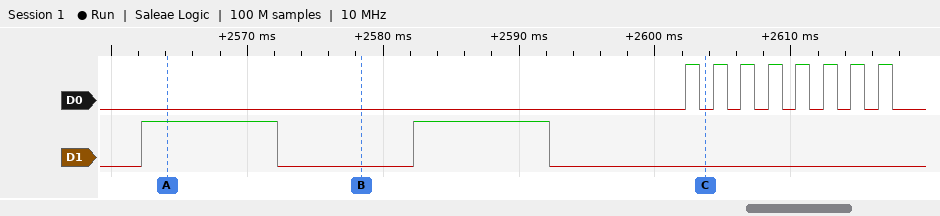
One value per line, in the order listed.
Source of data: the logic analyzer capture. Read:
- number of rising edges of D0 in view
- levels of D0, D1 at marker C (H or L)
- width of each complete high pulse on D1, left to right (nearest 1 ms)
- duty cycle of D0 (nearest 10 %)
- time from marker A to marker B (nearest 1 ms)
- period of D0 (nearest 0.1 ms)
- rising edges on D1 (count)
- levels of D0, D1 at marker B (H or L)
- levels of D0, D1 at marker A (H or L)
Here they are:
8
D0=L, D1=L
10 ms, 10 ms
50 %
14 ms
2 ms
2
D0=L, D1=L
D0=L, D1=H
